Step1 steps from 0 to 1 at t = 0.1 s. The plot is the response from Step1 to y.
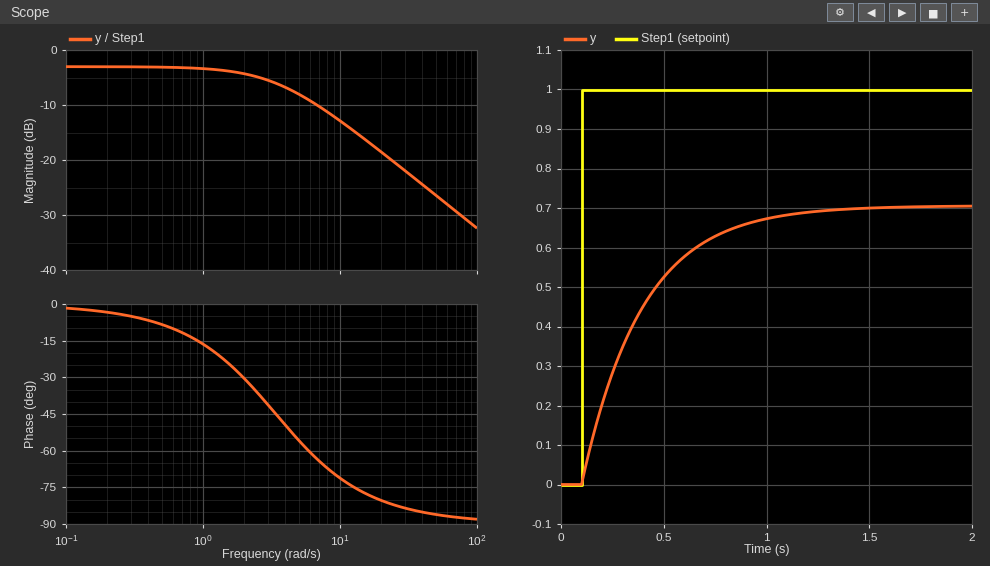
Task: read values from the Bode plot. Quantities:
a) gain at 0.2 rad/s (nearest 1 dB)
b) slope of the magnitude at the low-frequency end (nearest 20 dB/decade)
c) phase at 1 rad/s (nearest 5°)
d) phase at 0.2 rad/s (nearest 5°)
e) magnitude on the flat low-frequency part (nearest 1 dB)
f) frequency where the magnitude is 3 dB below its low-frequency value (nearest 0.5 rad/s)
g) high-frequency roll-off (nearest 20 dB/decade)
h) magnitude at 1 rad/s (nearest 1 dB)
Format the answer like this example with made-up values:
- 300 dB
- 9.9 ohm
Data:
- -3 dB
- 0 dB/decade
- -15°
- -5°
- -3 dB
- 3.5 rad/s
- -20 dB/decade
- -3 dB
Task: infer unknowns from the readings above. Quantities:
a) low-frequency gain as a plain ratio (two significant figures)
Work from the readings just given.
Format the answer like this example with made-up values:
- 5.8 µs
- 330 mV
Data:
- 0.71
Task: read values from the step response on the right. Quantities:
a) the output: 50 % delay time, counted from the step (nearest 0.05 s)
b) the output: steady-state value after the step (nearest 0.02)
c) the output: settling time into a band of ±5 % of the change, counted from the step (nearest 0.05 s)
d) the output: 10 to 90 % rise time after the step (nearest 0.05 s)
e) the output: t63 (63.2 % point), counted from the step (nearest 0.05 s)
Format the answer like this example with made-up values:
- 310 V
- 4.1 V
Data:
- 0.20 s
- 0.70
- 0.90 s
- 0.65 s
- 0.30 s
